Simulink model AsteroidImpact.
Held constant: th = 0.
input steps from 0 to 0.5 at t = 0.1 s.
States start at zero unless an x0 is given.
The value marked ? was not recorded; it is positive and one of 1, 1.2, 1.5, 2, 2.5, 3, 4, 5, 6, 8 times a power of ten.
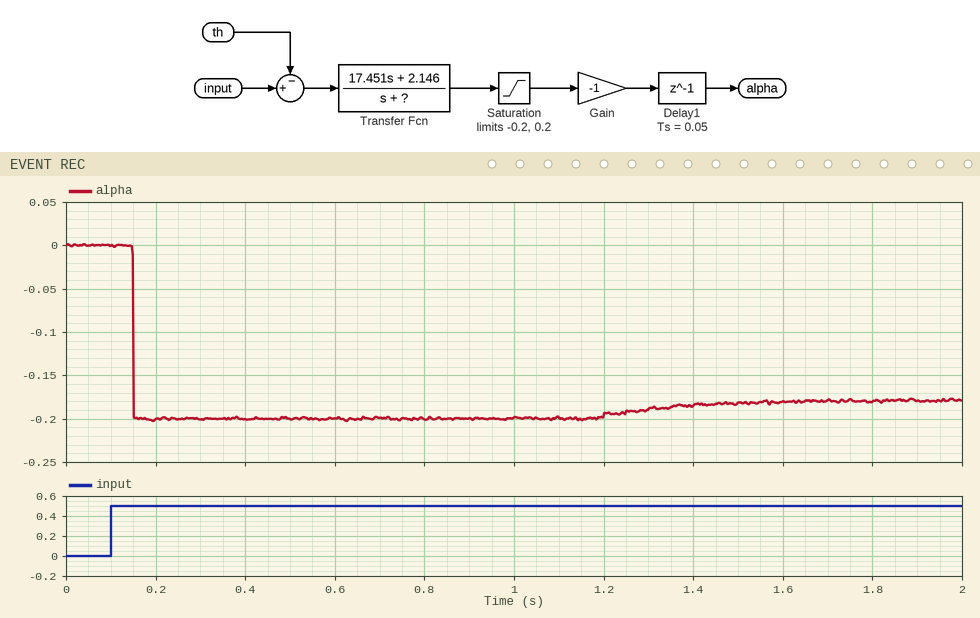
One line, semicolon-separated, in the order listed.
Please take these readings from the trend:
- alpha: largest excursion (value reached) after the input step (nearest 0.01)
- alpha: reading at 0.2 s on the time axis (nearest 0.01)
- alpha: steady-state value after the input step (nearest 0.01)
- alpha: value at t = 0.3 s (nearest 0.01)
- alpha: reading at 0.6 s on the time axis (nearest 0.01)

-0.20; -0.20; -0.18; -0.20; -0.20
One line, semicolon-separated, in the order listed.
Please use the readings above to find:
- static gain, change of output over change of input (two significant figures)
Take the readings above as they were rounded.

-0.36
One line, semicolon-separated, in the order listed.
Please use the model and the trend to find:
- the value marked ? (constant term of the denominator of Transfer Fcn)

6
